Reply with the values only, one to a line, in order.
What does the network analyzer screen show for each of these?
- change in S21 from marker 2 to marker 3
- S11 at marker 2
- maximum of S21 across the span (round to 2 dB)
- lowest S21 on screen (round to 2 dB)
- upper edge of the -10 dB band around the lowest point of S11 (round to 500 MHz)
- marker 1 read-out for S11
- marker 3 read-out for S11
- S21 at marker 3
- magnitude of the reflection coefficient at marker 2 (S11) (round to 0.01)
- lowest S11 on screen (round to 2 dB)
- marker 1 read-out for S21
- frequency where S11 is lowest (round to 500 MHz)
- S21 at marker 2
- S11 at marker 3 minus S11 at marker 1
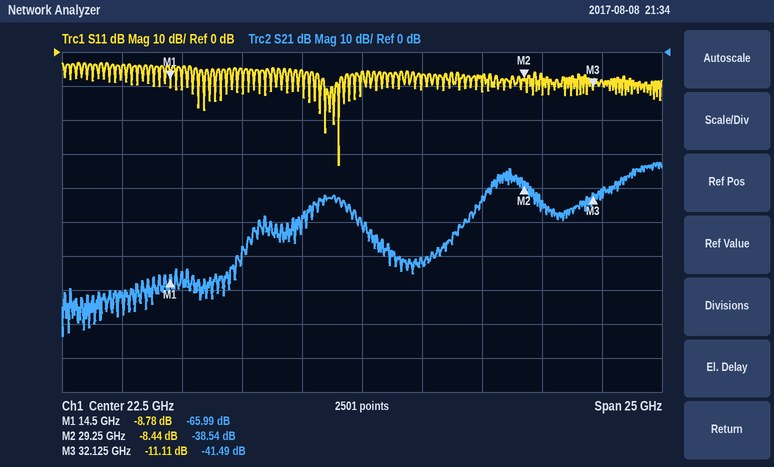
-2.95 dB
-8.44 dB
-32 dB
-84 dB
21.5 GHz
-8.78 dB
-11.11 dB
-41.49 dB
0.38
-34 dB
-65.99 dB
21.5 GHz
-38.54 dB
-2.33 dB
